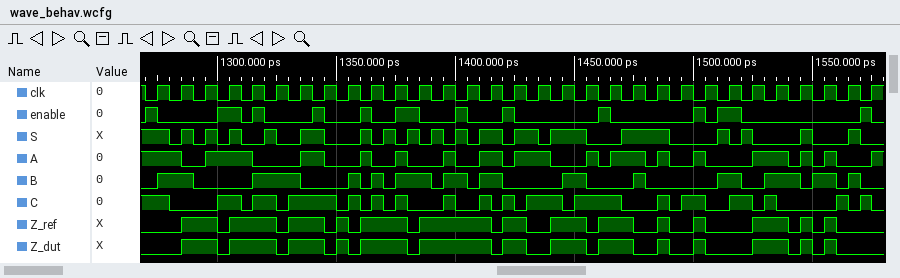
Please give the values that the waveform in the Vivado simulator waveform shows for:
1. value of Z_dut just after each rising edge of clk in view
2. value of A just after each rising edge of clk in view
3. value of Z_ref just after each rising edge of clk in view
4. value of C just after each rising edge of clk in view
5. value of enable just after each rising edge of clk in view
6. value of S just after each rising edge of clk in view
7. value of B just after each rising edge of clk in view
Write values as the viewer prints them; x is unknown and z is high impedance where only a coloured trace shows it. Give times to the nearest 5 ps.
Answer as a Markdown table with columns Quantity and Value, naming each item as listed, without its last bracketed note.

| Quantity | Value |
|---|---|
| value of Z_dut just after each rising edge of clk in view | 0 1 1 1 1 0 1 0 0 1 1 1 1 1 0 1 0 1 0 1 0 1 0 0 0 1 1 1 1 0 0 |
| value of A just after each rising edge of clk in view | 1 0 1 1 0 0 1 0 0 0 1 0 1 0 1 1 1 0 1 1 1 1 0 0 0 1 1 1 1 0 1 |
| value of Z_ref just after each rising edge of clk in view | 0 1 1 1 1 0 1 0 0 1 1 1 1 1 0 1 0 1 0 1 0 1 0 0 0 1 1 1 1 0 0 |
| value of C just after each rising edge of clk in view | 1 0 0 1 1 0 1 1 1 1 1 0 1 0 0 0 1 0 1 1 0 1 1 0 1 0 0 0 0 0 0 |
| value of enable just after each rising edge of clk in view | 0 0 0 1 1 0 0 0 0 0 1 0 0 0 0 0 0 0 0 0 0 0 0 0 1 0 0 0 0 0 0 |
| value of S just after each rising edge of clk in view | 1 1 1 1 0 0 1 0 0 0 0 0 0 0 1 1 0 1 0 0 1 1 0 0 0 0 0 1 0 1 0 |
| value of B just after each rising edge of clk in view | 1 1 0 0 1 1 0 0 1 1 1 1 1 0 1 0 0 1 0 0 1 0 0 0 1 0 1 0 1 1 0 |
